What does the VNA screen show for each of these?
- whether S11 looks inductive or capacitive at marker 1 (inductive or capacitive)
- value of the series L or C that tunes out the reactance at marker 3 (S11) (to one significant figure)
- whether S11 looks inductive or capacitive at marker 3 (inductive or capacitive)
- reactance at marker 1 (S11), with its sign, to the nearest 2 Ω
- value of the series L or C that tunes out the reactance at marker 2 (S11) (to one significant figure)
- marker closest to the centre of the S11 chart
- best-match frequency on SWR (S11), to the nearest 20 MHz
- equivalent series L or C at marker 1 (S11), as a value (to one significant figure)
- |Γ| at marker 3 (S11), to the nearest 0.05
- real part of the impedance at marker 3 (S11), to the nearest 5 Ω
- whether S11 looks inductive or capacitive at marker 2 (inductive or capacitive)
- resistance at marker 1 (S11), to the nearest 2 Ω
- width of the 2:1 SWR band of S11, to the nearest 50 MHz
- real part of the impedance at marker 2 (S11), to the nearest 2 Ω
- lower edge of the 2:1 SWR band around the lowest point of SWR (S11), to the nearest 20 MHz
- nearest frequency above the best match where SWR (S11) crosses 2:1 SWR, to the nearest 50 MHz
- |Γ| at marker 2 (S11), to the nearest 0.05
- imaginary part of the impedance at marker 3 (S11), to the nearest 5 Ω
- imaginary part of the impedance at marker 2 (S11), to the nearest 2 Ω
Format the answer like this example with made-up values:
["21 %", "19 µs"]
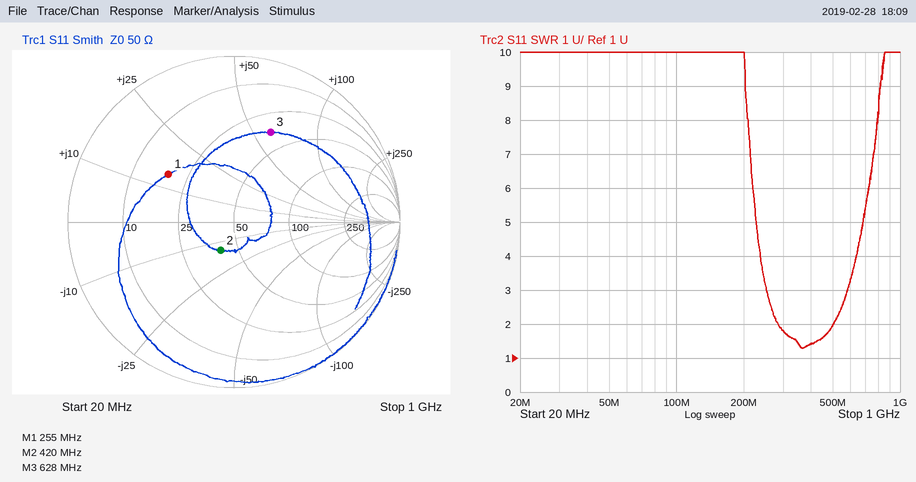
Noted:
["inductive", "4 pF", "inductive", "+14 Ω", "5 nH", "marker 2", "360 MHz", "9 nH", "0.60", "35 Ω", "capacitive", "18 Ω", "200 MHz", "40 Ω", "280 MHz", "500 MHz", "0.20", "+60 Ω", "-14 Ω"]
